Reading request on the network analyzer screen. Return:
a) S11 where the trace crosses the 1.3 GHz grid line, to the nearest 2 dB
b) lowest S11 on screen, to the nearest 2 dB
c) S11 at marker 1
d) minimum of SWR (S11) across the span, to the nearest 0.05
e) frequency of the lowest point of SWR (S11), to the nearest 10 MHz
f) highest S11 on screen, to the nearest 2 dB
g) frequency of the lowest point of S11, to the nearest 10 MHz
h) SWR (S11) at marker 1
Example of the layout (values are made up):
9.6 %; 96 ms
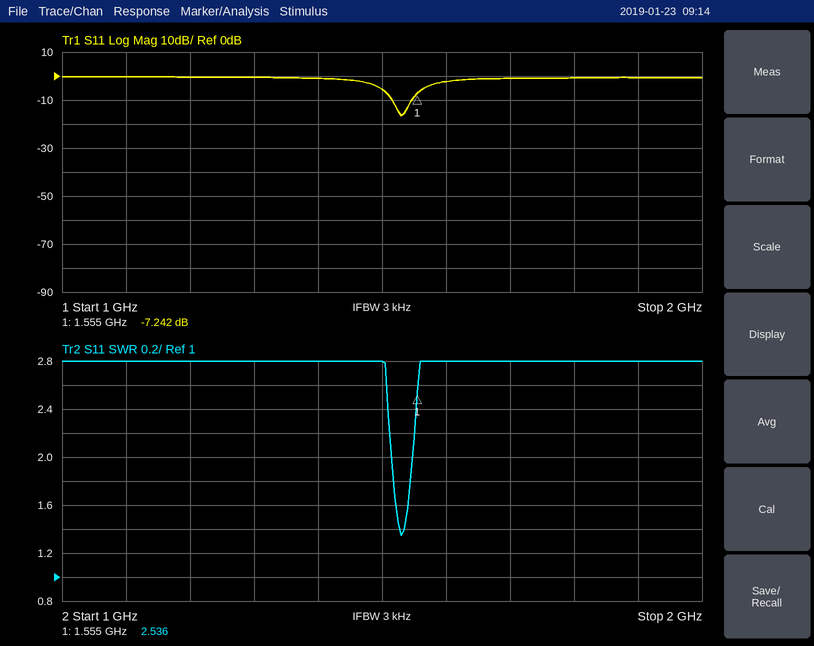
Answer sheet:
0 dB; -16 dB; -7.242 dB; 1.35; 1.53 GHz; 0 dB; 1.53 GHz; 2.536
